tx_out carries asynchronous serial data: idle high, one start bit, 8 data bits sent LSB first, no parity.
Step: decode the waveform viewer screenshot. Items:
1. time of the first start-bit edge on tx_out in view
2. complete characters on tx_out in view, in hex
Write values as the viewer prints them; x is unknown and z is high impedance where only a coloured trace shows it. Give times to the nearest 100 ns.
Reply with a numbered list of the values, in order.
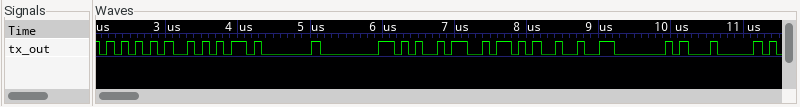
1. 2100 ns
2. 55, AA, 01, 80, A5, 5A, 92, 40, 04
